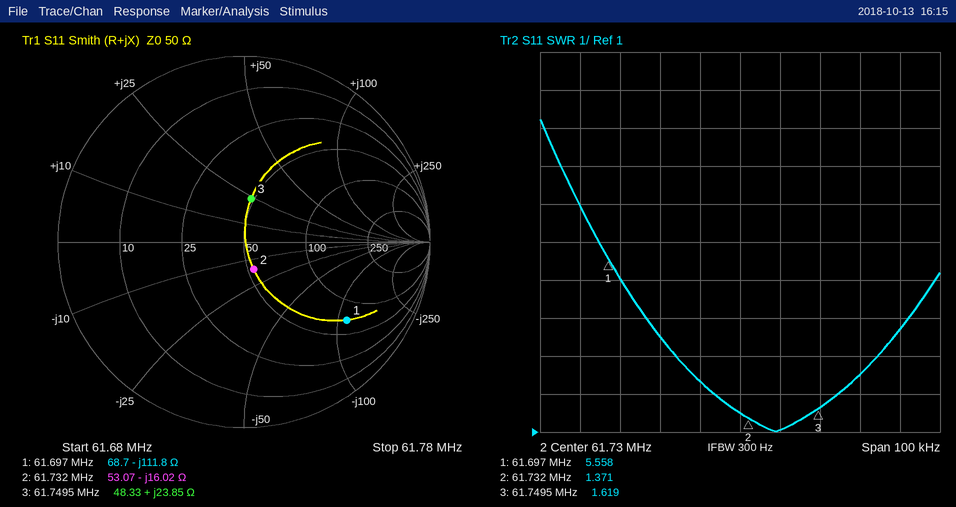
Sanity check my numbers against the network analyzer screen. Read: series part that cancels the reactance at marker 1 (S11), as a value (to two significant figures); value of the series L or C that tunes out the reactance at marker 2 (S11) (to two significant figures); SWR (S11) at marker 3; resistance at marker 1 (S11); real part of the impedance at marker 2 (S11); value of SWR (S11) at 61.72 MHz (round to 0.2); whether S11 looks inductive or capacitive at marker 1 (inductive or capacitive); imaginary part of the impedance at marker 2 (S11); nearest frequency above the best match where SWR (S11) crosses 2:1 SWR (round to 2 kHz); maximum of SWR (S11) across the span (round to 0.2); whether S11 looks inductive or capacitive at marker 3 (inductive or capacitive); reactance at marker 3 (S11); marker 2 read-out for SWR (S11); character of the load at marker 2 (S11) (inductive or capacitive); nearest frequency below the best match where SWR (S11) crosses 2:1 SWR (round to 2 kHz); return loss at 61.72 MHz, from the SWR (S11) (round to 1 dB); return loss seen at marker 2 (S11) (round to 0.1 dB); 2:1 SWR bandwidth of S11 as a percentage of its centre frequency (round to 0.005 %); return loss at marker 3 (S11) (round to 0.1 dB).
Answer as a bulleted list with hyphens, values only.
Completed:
- 290 nH
- 41 nH
- 1.619
- 68.7 Ω
- 53.07 Ω
- 2.4
- capacitive
- -16.02 Ω
- 61.754 MHz
- 9.2
- inductive
- +23.85 Ω
- 1.371
- capacitive
- 61.724 MHz
- 8 dB
- 16.1 dB
- 0.050 %
- 12.5 dB
